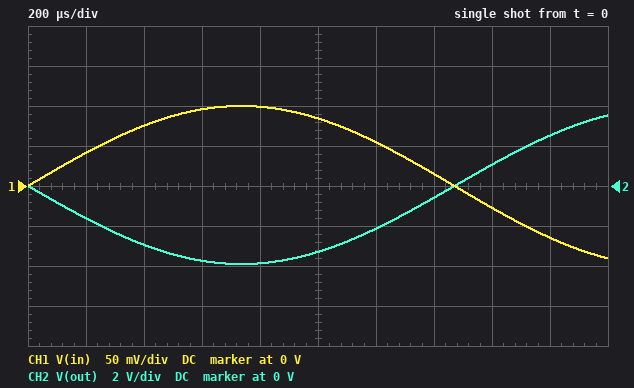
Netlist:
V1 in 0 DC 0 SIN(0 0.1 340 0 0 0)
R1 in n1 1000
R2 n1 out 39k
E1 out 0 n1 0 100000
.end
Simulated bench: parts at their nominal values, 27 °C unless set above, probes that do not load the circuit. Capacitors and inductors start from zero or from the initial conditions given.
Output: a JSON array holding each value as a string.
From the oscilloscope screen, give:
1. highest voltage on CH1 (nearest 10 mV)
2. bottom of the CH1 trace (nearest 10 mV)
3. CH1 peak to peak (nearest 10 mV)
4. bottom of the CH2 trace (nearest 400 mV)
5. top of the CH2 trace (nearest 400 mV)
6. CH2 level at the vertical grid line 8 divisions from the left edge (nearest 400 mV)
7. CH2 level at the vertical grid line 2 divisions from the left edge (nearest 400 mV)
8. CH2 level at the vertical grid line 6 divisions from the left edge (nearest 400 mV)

["100 mV", "-90 mV", "190 mV", "-4.0 V", "3.6 V", "1.2 V", "-2.8 V", "-2.0 V"]
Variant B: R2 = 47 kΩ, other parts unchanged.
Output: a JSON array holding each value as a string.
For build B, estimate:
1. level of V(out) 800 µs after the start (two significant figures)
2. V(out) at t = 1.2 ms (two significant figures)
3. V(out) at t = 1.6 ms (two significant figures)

["-4.7 V", "-2.6 V", "1.3 V"]
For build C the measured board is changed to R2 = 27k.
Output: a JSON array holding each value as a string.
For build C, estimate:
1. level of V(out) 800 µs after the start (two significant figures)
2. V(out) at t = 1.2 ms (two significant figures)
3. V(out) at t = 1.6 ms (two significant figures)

["-2.7 V", "-1.5 V", "740 mV"]
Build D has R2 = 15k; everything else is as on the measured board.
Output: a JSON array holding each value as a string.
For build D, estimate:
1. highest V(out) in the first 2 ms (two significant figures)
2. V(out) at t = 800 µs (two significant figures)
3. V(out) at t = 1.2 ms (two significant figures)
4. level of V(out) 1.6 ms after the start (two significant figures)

["1.4 V", "-1.5 V", "-820 mV", "410 mV"]
